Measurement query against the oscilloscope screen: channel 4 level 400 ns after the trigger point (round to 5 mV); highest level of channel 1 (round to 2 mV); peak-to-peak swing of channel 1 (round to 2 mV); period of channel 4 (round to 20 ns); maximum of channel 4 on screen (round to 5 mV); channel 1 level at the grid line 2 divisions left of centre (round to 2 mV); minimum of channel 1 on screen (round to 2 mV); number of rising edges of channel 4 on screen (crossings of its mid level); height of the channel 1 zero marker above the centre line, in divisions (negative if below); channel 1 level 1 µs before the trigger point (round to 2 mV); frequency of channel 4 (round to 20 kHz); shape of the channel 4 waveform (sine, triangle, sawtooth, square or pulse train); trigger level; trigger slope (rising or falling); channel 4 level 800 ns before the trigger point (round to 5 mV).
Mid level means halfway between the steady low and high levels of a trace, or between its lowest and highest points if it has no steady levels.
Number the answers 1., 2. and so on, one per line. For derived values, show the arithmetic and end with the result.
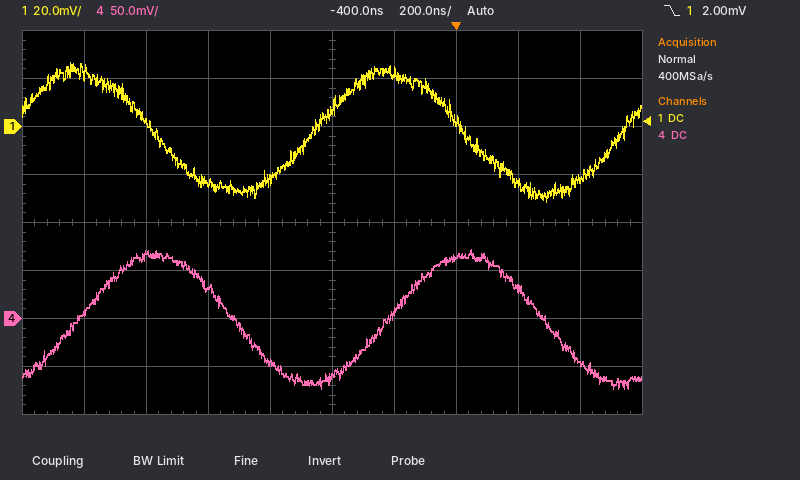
1. -45 mV
2. 26 mV
3. 26 mV − (-32 mV) = 58 mV
4. 1.00 µs
5. 70 mV
6. -24 mV
7. -32 mV
8. 2
9. +2.0 div
10. 2 mV
11. 1 / 1.00 µs ≈ 1.00 MHz
12. sine
13. 2.00 mV
14. falling
15. 30 mV
